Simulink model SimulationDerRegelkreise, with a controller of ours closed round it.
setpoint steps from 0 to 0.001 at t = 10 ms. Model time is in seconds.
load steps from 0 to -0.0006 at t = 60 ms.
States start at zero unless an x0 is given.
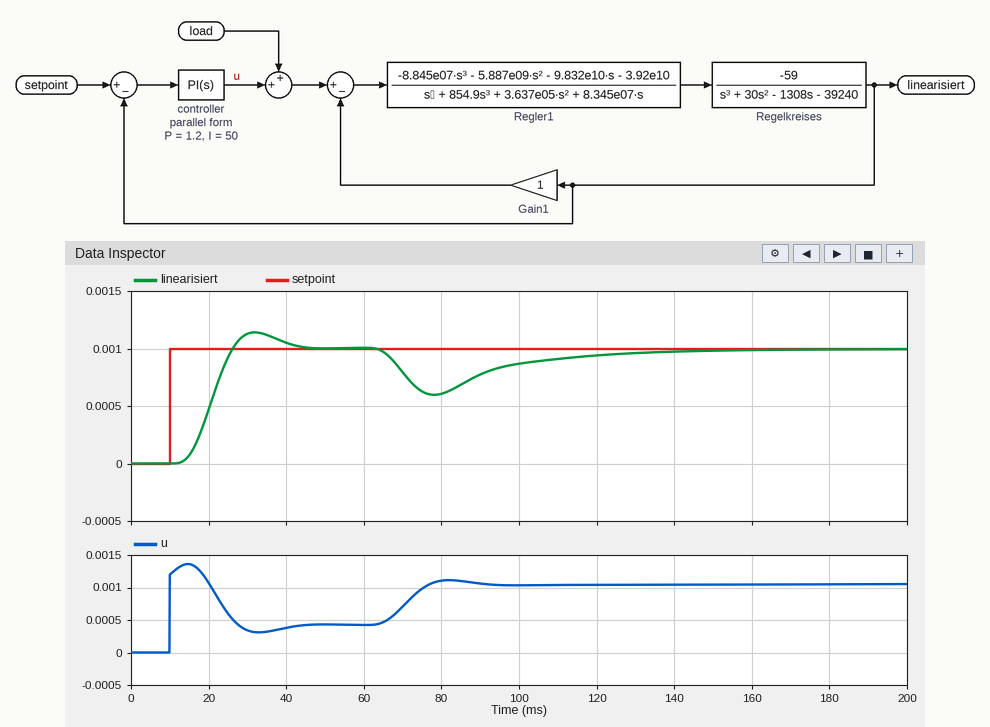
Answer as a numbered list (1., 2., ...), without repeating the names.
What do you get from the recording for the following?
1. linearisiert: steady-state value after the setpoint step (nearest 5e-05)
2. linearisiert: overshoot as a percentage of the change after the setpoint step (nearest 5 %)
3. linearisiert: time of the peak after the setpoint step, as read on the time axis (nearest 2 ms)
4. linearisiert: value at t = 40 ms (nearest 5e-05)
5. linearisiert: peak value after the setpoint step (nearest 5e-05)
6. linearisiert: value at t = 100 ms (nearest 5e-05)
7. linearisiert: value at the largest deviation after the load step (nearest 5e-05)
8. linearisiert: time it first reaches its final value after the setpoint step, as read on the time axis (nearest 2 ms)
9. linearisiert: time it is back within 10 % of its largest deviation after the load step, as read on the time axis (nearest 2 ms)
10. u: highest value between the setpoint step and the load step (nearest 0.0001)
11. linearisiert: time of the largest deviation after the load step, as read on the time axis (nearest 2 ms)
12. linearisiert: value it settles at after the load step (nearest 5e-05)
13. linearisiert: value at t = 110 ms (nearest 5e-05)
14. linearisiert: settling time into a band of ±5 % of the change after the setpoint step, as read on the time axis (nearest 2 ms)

1. 0.00100
2. 15 %
3. 32 ms
4. 0.00105
5. 0.00115
6. 0.00085
7. 0.00060
8. 26 ms
9. 128 ms
10. 0.0014
11. 78 ms
12. 0.00100
13. 0.00090
14. 40 ms
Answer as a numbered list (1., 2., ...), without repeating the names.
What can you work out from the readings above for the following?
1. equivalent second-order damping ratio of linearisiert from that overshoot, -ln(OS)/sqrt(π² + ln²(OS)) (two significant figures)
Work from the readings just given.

1. 0.52
